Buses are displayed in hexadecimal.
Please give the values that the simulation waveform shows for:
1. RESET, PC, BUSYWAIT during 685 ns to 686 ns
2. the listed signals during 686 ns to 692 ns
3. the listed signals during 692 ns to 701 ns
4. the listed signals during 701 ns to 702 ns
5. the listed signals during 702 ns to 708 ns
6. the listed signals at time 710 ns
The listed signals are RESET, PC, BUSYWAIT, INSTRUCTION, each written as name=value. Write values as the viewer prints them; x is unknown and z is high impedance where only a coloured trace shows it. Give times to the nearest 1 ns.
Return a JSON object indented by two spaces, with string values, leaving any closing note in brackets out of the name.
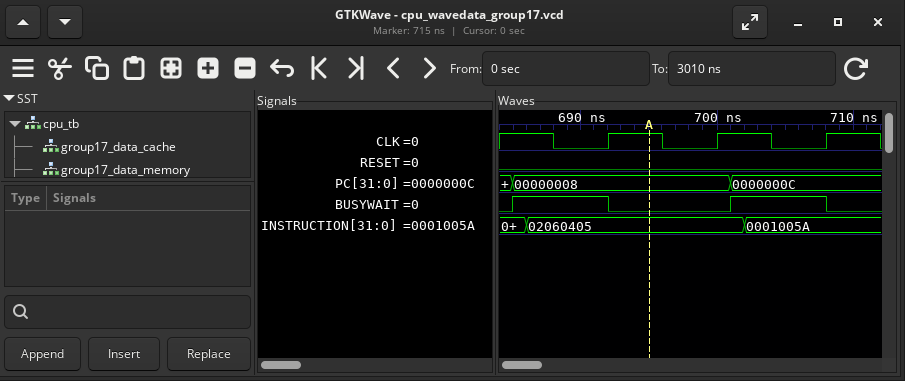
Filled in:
{
  "RESET, PC, BUSYWAIT during 685 ns to 686 ns": "RESET=0, PC=00000008, BUSYWAIT=1",
  "the listed signals during 686 ns to 692 ns": "RESET=0, PC=00000008, BUSYWAIT=1, INSTRUCTION=02060405",
  "the listed signals during 692 ns to 701 ns": "RESET=0, PC=00000008, BUSYWAIT=0, INSTRUCTION=02060405",
  "the listed signals during 701 ns to 702 ns": "RESET=0, PC=0000000C, BUSYWAIT=1, INSTRUCTION=02060405",
  "the listed signals during 702 ns to 708 ns": "RESET=0, PC=0000000C, BUSYWAIT=1, INSTRUCTION=0001005A",
  "the listed signals at time 710 ns": "RESET=0, PC=0000000C, BUSYWAIT=0, INSTRUCTION=0001005A"
}
